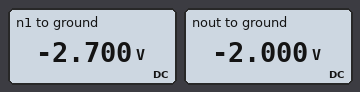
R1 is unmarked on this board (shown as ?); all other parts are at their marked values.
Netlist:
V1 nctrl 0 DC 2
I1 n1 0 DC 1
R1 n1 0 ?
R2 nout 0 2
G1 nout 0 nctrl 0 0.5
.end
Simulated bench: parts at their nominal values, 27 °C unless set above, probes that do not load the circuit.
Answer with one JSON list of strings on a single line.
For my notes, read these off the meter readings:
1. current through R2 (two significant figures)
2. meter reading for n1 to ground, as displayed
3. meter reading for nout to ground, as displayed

["1.0 A", "-2.700 V", "-2.000 V"]
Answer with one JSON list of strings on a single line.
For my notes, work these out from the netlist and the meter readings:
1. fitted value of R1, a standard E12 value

["2.7 Ω"]
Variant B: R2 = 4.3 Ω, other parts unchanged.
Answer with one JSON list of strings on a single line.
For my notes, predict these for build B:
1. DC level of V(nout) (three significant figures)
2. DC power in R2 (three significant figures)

["-4.30 V", "4.30 W"]
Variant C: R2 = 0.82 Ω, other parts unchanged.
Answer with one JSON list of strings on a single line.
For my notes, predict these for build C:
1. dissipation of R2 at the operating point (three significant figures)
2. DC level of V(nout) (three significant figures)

["820 mW", "-820 mV"]
